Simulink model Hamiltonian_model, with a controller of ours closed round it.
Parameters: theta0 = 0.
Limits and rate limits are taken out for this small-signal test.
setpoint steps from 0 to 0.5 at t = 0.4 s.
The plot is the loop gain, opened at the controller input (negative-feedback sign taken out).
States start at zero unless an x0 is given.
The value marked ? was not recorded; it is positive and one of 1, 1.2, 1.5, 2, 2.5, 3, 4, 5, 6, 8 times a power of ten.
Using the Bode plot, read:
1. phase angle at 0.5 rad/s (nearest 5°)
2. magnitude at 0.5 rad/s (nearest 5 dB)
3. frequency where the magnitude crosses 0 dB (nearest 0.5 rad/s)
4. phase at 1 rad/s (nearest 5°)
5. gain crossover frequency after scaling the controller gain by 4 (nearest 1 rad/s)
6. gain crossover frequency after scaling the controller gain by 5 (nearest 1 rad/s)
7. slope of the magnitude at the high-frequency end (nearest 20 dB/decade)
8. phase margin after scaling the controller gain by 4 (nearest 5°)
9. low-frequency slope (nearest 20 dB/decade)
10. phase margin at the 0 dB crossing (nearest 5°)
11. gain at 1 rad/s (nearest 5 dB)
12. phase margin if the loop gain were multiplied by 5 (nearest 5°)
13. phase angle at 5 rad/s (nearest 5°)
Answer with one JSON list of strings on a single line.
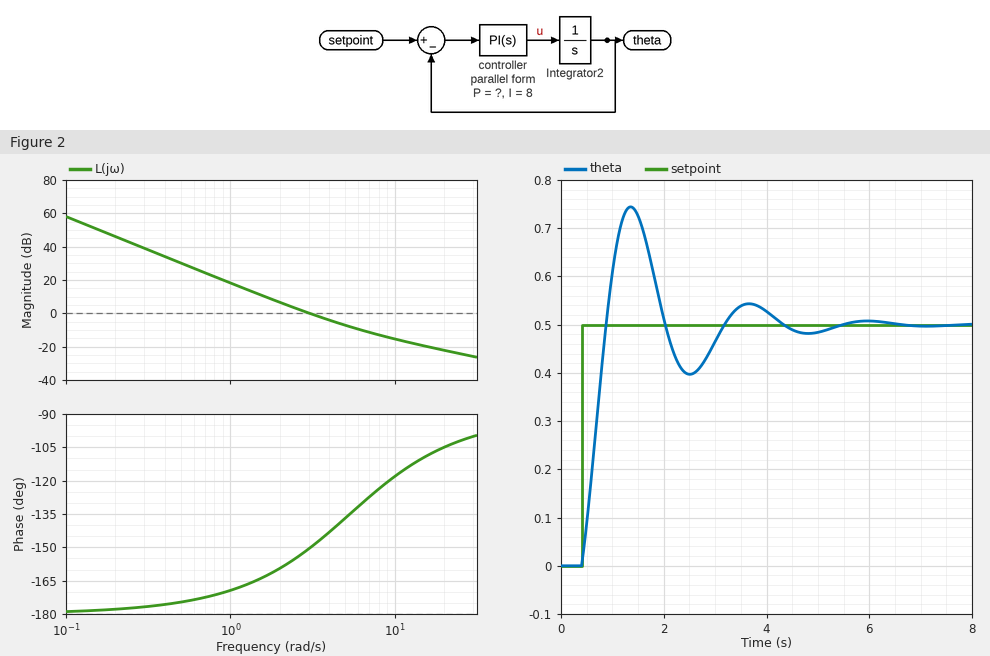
["-175°", "30 dB", "3.0 rad/s", "-170°", "7 rad/s", "9 rad/s", "-20 dB/decade", "55°", "-40 dB/decade", "30°", "20 dB", "60°", "-135°"]
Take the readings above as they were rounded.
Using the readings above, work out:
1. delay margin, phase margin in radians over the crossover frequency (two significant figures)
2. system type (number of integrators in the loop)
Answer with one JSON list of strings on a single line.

["0.17 s", "2"]
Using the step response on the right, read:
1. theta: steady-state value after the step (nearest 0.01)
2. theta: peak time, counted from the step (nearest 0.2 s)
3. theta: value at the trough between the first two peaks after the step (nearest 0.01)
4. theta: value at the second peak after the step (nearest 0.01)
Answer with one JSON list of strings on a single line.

["0.50", "1.0 s", "0.40", "0.54"]
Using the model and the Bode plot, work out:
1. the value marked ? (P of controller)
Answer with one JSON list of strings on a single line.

["1.5"]
